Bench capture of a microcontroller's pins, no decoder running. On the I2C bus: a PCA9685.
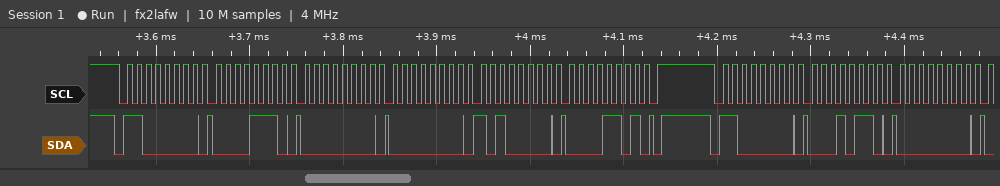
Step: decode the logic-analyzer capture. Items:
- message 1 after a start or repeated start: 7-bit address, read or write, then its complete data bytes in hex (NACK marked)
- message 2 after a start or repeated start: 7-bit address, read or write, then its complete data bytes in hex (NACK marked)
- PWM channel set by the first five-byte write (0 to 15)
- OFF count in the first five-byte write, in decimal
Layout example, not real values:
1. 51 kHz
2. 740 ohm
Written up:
1. 0x60 write: 0E 00 00 A0 0D
2. 0x60 write: 16 00
3. 2
4. 3488
